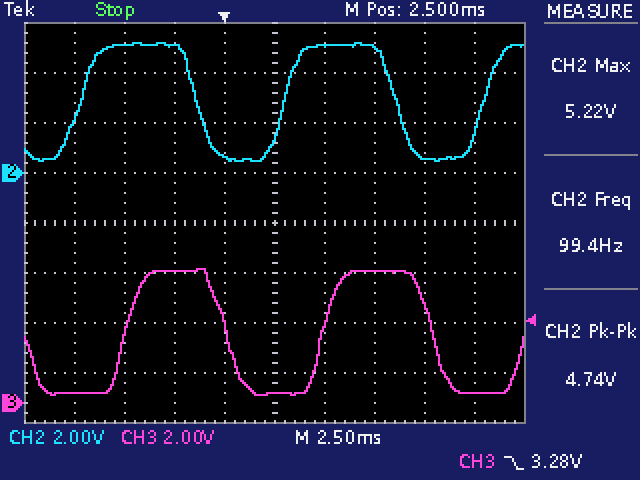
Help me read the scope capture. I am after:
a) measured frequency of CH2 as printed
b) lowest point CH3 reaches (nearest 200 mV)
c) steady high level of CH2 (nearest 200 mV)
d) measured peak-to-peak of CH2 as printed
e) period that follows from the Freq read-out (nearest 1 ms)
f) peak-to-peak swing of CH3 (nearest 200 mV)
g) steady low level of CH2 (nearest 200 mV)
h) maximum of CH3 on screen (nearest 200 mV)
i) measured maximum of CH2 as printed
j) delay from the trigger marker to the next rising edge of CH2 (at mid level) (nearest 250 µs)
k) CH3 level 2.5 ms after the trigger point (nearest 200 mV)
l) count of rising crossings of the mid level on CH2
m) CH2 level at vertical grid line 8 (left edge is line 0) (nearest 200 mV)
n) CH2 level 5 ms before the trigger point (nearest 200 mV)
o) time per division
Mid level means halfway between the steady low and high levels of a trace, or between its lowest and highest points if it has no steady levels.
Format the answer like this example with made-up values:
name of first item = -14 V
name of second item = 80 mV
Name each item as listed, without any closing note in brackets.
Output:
measured frequency of CH2 as printed = 99.4 Hz
lowest point CH3 reaches = 400 mV
steady high level of CH2 = 5.2 V
measured peak-to-peak of CH2 as printed = 4.74 V
period that follows from the Freq read-out = 10 ms
peak-to-peak swing of CH3 = 5.0 V
steady low level of CH2 = 600 mV
maximum of CH3 on screen = 5.4 V
measured maximum of CH2 as printed = 5.22 V
delay from the trigger marker to the next rising edge of CH2 (at mid level) = 3.00 ms
CH3 level 2.5 ms after the trigger point = 400 mV
count of rising crossings of the mid level on CH2 = 3
CH2 level at vertical grid line 8 (left edge is line 0) = 600 mV
CH2 level 5 ms before the trigger point = 5.2 V
time per division = 2.5 ms
